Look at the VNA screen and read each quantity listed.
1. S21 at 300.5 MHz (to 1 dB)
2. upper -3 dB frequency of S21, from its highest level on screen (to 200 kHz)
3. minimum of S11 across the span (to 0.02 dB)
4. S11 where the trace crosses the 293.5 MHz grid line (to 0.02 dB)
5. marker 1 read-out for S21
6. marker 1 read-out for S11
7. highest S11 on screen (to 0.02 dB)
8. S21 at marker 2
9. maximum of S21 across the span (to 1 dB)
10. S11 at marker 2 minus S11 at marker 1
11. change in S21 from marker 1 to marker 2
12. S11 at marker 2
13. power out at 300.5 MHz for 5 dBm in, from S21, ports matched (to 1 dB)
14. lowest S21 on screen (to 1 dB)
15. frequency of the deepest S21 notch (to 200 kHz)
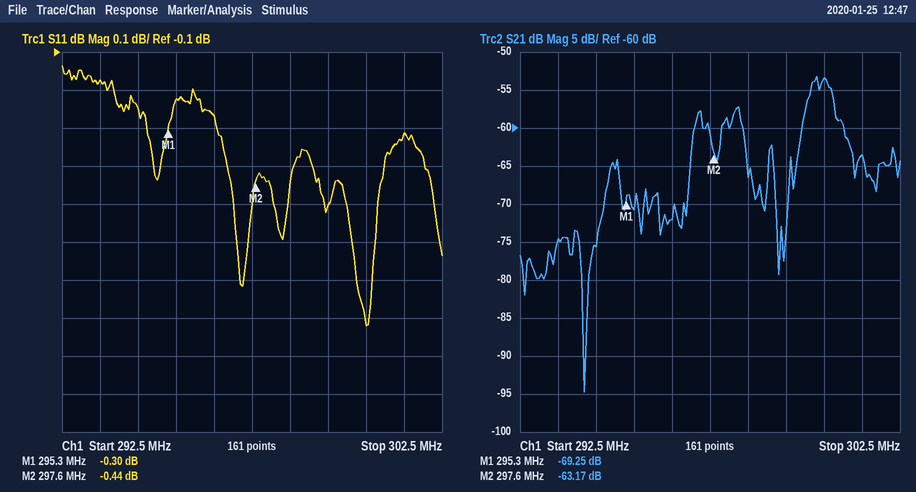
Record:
-53 dB
300.8 MHz
-0.82 dB
-0.18 dB
-69.25 dB
-0.30 dB
-0.14 dB
-63.17 dB
-53 dB
-0.14 dB
6.08 dB
-0.44 dB
-48 dBm
-95 dB
294.2 MHz
